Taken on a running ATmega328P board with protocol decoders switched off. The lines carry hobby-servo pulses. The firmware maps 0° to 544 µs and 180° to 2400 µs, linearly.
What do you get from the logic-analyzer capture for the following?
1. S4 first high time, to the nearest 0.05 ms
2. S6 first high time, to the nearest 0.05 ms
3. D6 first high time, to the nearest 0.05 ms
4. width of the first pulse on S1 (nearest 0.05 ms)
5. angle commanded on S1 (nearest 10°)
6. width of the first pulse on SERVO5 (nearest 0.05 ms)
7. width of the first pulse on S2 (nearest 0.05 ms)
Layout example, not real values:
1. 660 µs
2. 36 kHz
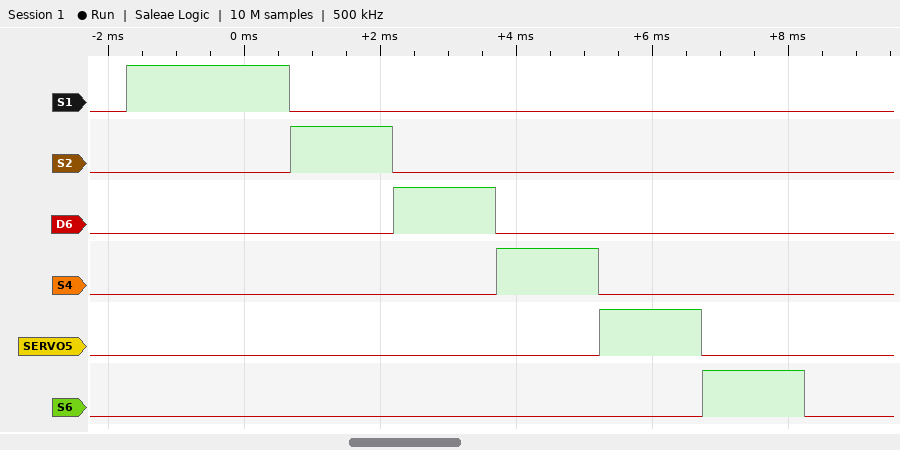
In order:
1. 1.50 ms
2. 1.50 ms
3. 1.50 ms
4. 2.40 ms
5. 180°
6. 1.50 ms
7. 1.50 ms
